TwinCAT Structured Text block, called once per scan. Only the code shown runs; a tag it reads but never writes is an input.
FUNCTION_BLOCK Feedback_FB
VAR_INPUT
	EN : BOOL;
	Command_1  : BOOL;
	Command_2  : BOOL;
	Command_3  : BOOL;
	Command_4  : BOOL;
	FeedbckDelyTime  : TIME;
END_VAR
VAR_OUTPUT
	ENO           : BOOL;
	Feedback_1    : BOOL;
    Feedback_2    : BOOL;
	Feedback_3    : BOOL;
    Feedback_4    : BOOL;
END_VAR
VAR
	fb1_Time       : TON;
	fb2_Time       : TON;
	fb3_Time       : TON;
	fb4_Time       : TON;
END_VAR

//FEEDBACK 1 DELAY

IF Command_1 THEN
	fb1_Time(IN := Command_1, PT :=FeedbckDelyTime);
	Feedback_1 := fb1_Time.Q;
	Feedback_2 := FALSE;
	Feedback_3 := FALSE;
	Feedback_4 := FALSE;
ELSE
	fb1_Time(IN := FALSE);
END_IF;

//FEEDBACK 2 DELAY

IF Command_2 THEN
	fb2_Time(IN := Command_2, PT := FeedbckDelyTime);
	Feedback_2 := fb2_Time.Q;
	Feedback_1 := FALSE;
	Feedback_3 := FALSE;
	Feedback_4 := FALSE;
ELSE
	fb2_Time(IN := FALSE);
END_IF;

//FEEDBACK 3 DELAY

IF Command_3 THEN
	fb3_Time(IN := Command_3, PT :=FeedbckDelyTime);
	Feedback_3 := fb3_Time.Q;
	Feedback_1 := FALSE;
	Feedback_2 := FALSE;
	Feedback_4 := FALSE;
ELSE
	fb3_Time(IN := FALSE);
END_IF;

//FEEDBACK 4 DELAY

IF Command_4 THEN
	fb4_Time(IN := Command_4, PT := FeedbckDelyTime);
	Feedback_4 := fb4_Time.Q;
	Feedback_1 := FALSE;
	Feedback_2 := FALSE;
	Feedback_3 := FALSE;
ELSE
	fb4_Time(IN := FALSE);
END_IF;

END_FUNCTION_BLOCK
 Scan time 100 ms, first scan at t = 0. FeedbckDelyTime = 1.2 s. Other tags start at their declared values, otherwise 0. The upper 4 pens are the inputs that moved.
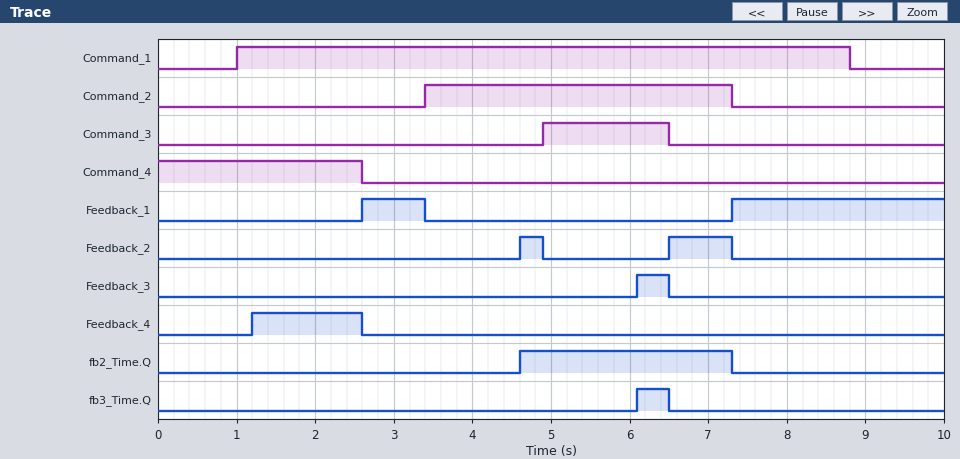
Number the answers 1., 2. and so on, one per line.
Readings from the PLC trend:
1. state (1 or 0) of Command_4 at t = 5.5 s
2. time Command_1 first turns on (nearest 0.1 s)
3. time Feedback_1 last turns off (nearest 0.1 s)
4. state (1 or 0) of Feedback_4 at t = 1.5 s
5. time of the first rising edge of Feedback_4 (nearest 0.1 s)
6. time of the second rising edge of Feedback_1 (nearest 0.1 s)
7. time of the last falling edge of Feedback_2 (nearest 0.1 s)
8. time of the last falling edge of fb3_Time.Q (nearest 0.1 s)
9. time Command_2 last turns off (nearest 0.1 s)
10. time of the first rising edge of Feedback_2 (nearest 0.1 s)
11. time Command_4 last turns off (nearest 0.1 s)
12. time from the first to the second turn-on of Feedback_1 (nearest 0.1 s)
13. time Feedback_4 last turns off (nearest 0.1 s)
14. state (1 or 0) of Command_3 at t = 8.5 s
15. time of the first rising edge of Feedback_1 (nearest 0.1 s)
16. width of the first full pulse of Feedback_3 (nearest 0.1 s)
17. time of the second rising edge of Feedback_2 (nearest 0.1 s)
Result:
1. 0
2. 1.0 s
3. 3.4 s
4. 1
5. 1.2 s
6. 7.3 s
7. 7.3 s
8. 6.5 s
9. 7.3 s
10. 4.6 s
11. 2.6 s
12. 4.7 s
13. 2.6 s
14. 0
15. 2.6 s
16. 0.4 s
17. 6.5 s
